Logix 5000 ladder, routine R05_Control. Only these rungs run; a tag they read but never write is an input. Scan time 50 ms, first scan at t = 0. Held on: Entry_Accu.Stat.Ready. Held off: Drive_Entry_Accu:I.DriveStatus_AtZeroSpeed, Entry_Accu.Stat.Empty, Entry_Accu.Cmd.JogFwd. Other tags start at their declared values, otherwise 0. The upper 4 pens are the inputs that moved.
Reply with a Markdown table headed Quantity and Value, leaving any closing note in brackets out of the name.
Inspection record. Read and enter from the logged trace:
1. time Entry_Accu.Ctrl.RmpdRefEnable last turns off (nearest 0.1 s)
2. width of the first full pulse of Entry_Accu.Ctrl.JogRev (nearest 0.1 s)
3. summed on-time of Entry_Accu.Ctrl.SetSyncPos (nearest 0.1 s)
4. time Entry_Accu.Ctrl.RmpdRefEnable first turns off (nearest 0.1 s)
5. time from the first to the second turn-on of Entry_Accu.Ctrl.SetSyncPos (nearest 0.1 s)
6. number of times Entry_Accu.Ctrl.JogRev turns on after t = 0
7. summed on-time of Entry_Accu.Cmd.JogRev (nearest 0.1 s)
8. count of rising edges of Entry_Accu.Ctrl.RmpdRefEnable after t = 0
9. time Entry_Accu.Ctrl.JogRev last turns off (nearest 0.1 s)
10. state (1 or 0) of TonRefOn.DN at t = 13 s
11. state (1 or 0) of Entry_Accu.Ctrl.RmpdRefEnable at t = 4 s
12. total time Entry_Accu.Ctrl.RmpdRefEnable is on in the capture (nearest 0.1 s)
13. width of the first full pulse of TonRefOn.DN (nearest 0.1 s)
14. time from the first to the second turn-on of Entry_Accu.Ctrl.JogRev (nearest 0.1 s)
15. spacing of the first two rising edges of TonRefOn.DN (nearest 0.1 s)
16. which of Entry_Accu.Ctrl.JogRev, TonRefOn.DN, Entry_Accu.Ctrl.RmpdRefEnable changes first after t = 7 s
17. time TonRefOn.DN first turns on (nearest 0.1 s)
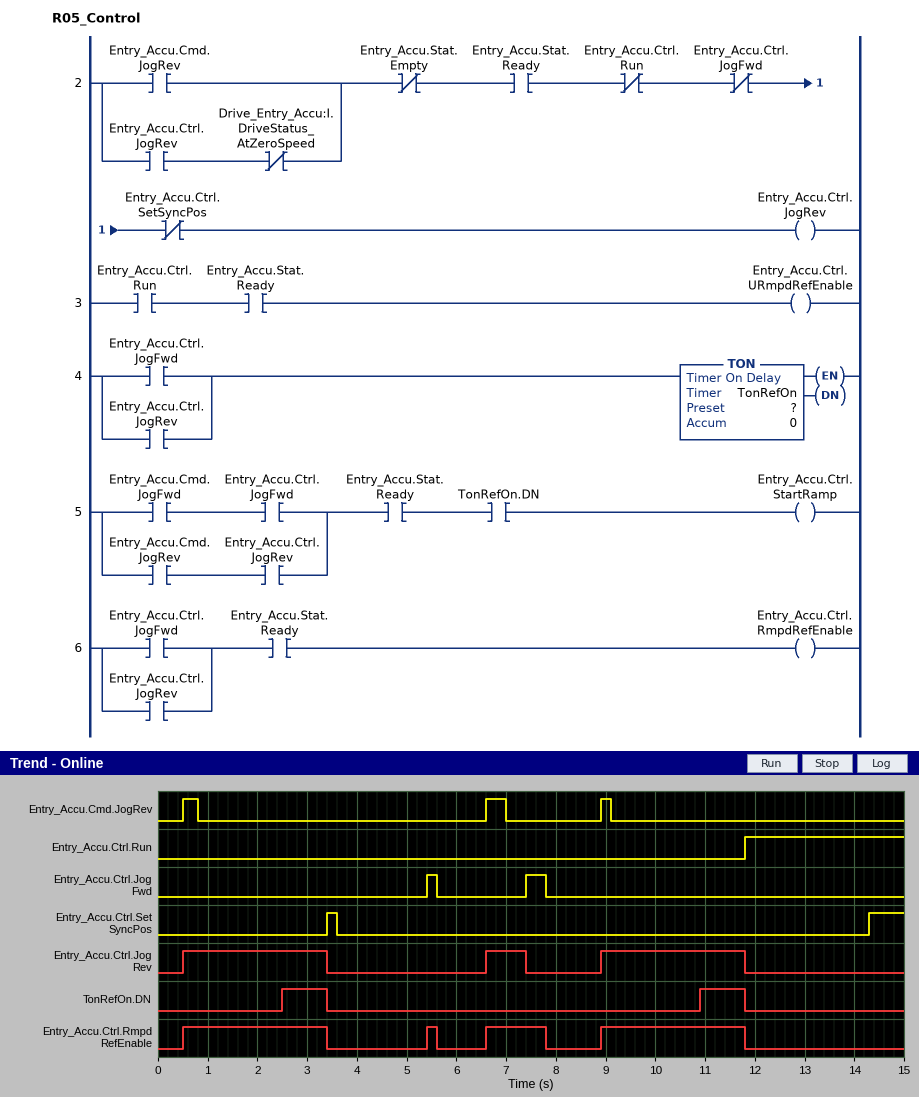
| Quantity | Value |
|---|---|
| time Entry_Accu.Ctrl.RmpdRefEnable last turns off | 11.8 s |
| width of the first full pulse of Entry_Accu.Ctrl.JogRev | 2.9 s |
| summed on-time of Entry_Accu.Ctrl.SetSyncPos | 0.9 s |
| time Entry_Accu.Ctrl.RmpdRefEnable first turns off | 3.4 s |
| time from the first to the second turn-on of Entry_Accu.Ctrl.SetSyncPos | 10.9 s |
| number of times Entry_Accu.Ctrl.JogRev turns on after t = 0 | 3 |
| summed on-time of Entry_Accu.Cmd.JogRev | 0.9 s |
| count of rising edges of Entry_Accu.Ctrl.RmpdRefEnable after t = 0 | 4 |
| time Entry_Accu.Ctrl.JogRev last turns off | 11.8 s |
| state (1 or 0) of TonRefOn.DN at t = 13 s | 0 |
| state (1 or 0) of Entry_Accu.Ctrl.RmpdRefEnable at t = 4 s | 0 |
| total time Entry_Accu.Ctrl.RmpdRefEnable is on in the capture | 7.2 s |
| width of the first full pulse of TonRefOn.DN | 0.9 s |
| time from the first to the second turn-on of Entry_Accu.Ctrl.JogRev | 6.1 s |
| spacing of the first two rising edges of TonRefOn.DN | 8.4 s |
| which of Entry_Accu.Ctrl.JogRev, TonRefOn.DN, Entry_Accu.Ctrl.RmpdRefEnable changes first after t = 7 s | Entry_Accu.Ctrl.JogRev |
| time TonRefOn.DN first turns on | 2.5 s |
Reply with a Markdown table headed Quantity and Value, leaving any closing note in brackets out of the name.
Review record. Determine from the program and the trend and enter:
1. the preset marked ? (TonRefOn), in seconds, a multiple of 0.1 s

| Quantity | Value |
|---|---|
| the preset marked ? (TonRefOn), in seconds, a multiple of 0.1 s | 2.0 s |
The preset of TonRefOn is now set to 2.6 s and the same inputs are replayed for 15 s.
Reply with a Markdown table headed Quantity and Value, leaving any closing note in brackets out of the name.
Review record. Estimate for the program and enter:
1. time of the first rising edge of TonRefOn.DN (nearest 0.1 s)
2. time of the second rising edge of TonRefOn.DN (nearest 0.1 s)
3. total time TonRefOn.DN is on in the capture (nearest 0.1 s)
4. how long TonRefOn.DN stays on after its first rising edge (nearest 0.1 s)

| Quantity | Value |
|---|---|
| time of the first rising edge of TonRefOn.DN | 3.1 s |
| time of the second rising edge of TonRefOn.DN | 11.5 s |
| total time TonRefOn.DN is on in the capture | 0.6 s |
| how long TonRefOn.DN stays on after its first rising edge | 0.3 s |
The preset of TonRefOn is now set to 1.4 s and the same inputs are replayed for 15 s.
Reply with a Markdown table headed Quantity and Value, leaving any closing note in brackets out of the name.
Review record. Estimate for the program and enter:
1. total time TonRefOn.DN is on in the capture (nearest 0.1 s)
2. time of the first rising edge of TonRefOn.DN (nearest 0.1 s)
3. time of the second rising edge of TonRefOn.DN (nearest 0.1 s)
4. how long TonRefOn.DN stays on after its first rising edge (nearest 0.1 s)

| Quantity | Value |
|---|---|
| total time TonRefOn.DN is on in the capture | 3.0 s |
| time of the first rising edge of TonRefOn.DN | 1.9 s |
| time of the second rising edge of TonRefOn.DN | 10.3 s |
| how long TonRefOn.DN stays on after its first rising edge | 1.5 s |
